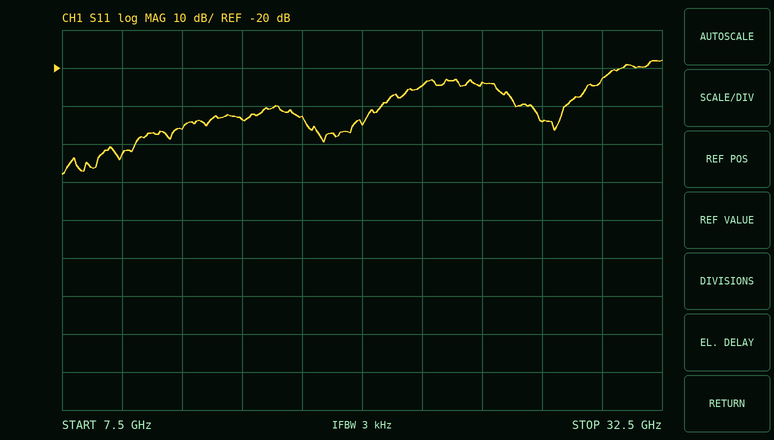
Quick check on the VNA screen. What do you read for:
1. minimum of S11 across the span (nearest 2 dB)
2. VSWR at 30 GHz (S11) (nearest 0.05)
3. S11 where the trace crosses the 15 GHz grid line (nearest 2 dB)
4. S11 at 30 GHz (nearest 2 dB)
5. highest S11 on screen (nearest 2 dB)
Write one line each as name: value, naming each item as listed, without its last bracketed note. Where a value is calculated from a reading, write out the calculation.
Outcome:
minimum of S11 across the span: -48 dB
VSWR at 30 GHz (S11): |Γ| = 10^(-22/20) = 0.0794; VSWR = (1 + 0.0794)/(1 − 0.0794) ≈ 1.17, so 1.15 to the nearest 0.05
S11 where the trace crosses the 15 GHz grid line: -34 dB
S11 at 30 GHz: -22 dB
highest S11 on screen: -18 dB
